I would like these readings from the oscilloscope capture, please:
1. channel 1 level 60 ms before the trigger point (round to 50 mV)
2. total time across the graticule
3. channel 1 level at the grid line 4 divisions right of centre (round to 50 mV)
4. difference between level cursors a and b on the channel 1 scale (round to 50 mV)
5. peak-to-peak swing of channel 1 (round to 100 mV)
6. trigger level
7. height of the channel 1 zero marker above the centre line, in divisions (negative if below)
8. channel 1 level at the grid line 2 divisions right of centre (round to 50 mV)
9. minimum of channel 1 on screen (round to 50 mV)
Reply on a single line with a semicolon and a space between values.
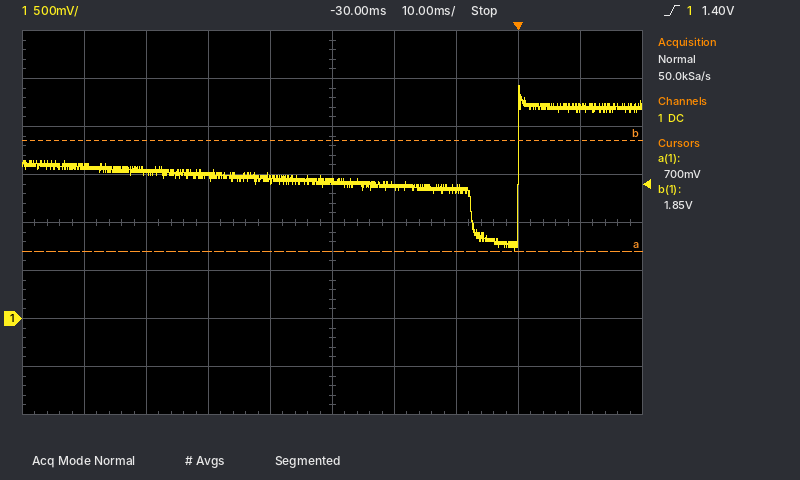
1.50 V; 100 ms; 2.20 V; 1.15 V; 1.70 V; 1.40 V; -2.0 div; 1.35 V; 700 mV
